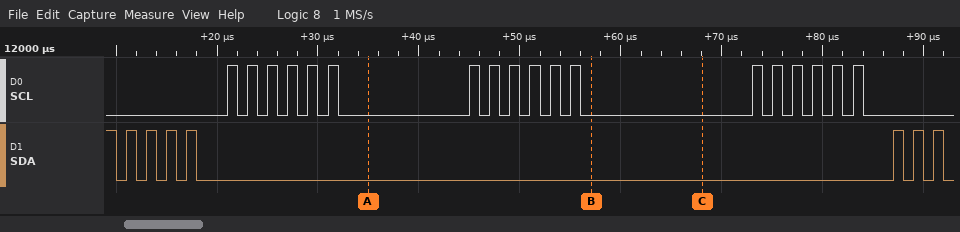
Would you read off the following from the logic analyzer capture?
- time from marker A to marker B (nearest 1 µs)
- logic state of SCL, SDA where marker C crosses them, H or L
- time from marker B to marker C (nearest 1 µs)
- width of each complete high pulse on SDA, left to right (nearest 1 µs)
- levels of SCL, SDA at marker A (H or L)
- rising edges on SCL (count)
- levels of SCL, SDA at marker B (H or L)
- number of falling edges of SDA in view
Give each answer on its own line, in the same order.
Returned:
22 µs
SCL=L, SDA=L
11 µs
1 µs, 1 µs, 1 µs, 1 µs, 1 µs, 1 µs, 1 µs
SCL=L, SDA=L
18
SCL=L, SDA=L
8
